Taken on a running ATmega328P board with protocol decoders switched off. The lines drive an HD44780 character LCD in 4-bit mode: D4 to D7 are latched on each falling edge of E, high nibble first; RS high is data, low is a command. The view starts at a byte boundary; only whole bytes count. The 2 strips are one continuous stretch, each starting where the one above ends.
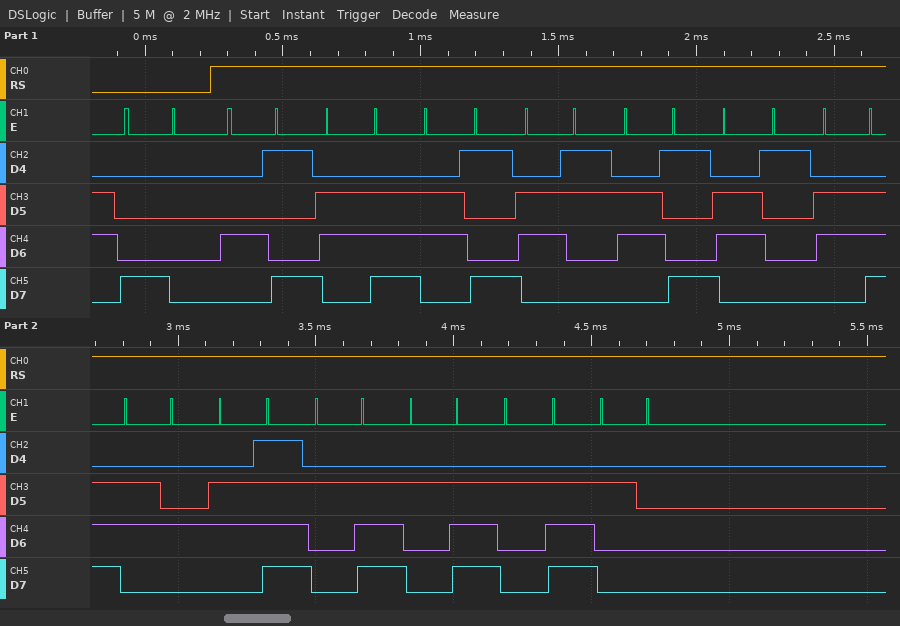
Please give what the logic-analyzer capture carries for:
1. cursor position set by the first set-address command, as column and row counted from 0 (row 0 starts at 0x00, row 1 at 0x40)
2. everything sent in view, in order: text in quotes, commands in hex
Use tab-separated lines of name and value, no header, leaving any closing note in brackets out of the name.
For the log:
cursor position set by the first set-address command, as column and row counted from 0	column 0, row 0
everything sent in view, in order: text in quotes, commands in hex	0x80 "Iniciando... "
